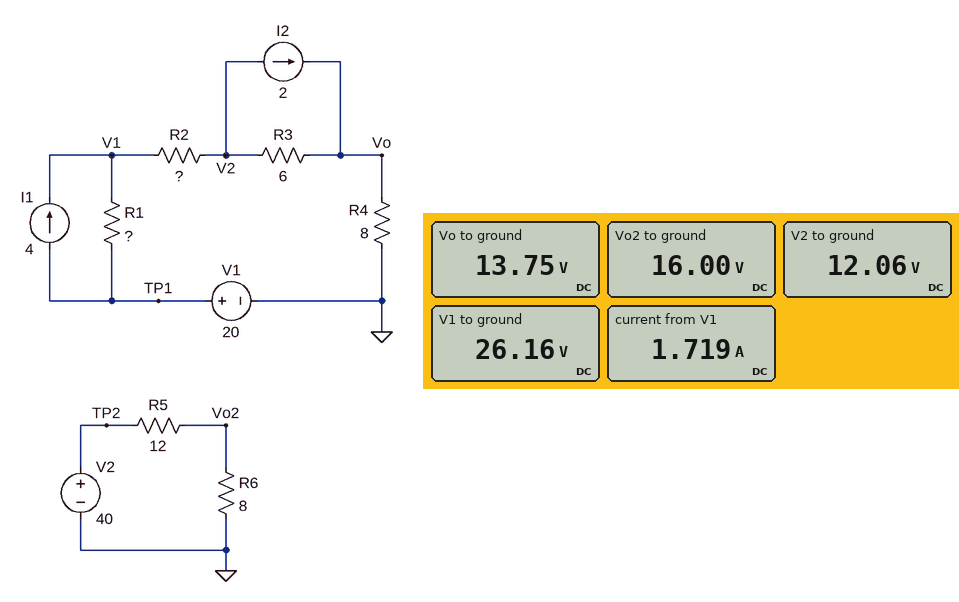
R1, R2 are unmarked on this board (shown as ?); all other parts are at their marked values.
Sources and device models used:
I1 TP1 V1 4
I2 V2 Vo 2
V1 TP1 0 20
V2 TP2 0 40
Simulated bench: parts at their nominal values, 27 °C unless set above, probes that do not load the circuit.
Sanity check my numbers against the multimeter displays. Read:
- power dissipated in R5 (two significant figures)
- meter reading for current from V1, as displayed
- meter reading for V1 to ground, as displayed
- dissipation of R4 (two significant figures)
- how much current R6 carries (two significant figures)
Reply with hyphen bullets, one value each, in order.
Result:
- 48 W
- 1.719 A
- 26.16 V
- 24 W
- 2.0 A
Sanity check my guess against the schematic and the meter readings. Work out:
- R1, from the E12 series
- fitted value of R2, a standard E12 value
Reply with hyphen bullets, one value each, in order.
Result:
- 2.7 Ω
- 8.2 Ω
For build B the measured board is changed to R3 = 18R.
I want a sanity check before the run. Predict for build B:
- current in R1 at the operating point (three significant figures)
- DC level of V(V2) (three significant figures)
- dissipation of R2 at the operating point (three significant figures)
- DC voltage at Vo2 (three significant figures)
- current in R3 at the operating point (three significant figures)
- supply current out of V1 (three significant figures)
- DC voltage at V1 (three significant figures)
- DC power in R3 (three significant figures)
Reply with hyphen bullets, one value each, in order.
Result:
- 2.19 A
- 11.1 V
- 26.9 W
- 16.0 V
- 190 mA
- 1.81 A
- 25.9 V
- 648 mW
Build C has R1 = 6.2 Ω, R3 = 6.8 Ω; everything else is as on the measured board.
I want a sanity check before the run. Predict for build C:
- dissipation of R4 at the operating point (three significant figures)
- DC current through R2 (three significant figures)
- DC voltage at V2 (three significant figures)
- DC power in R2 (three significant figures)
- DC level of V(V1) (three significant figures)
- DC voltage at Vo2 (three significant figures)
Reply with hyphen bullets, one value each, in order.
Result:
- 32.0 W
- 2.00 A
- 16.0 V
- 32.8 W
- 32.4 V
- 16.0 V
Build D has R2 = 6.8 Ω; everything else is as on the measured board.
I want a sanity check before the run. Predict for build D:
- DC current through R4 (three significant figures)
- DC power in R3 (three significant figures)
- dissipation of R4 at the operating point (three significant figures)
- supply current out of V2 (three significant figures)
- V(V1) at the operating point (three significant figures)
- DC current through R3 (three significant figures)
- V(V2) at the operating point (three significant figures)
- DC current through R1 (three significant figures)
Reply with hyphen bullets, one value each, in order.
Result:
- 1.82 A
- 192 mW
- 26.5 W
- 2.00 A
- 25.9 V
- 179 mA
- 13.5 V
- 2.18 A
